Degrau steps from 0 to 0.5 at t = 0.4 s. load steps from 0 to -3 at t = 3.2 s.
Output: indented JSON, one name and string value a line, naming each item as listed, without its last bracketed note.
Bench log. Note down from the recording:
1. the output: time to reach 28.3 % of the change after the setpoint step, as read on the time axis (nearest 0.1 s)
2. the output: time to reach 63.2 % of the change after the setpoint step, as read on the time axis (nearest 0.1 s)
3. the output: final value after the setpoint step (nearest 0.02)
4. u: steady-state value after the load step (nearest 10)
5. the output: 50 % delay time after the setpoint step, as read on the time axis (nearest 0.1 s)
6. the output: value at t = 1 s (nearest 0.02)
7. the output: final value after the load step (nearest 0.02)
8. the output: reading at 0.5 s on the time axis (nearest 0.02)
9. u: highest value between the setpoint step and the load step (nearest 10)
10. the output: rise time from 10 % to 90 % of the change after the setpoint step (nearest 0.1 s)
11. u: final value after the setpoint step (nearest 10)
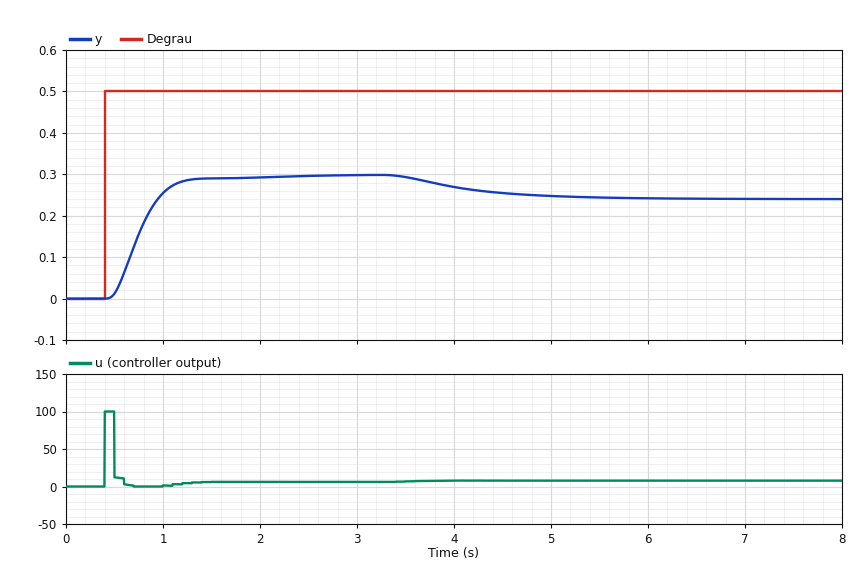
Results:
{
  "the output: time to reach 28.3 % of the change after the setpoint step, as read on the time axis": "0.6 s",
  "the output: time to reach 63.2 % of the change after the setpoint step, as read on the time axis": "0.8 s",
  "the output: final value after the setpoint step": "0.30",
  "u: steady-state value after the load step": "10",
  "the output: 50 % delay time after the setpoint step, as read on the time axis": "0.7 s",
  "the output: value at t = 1 s": "0.26",
  "the output: final value after the load step": "0.24",
  "the output: reading at 0.5 s on the time axis": "0.02",
  "u: highest value between the setpoint step and the load step": "100",
  "the output: rise time from 10 % to 90 % of the change after the setpoint step": "0.5 s",
  "u: final value after the setpoint step": "10"
}
